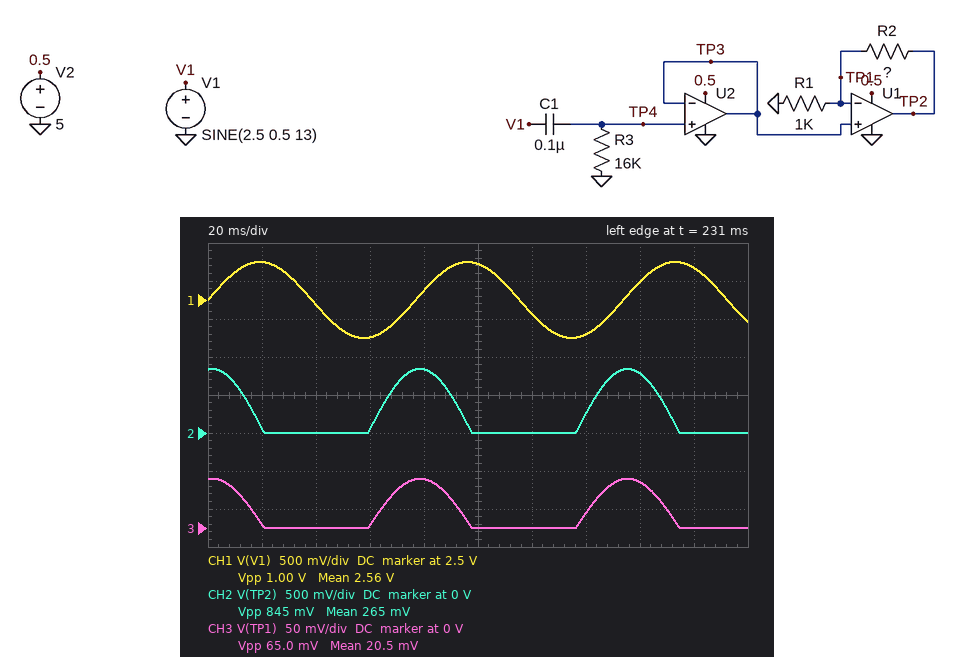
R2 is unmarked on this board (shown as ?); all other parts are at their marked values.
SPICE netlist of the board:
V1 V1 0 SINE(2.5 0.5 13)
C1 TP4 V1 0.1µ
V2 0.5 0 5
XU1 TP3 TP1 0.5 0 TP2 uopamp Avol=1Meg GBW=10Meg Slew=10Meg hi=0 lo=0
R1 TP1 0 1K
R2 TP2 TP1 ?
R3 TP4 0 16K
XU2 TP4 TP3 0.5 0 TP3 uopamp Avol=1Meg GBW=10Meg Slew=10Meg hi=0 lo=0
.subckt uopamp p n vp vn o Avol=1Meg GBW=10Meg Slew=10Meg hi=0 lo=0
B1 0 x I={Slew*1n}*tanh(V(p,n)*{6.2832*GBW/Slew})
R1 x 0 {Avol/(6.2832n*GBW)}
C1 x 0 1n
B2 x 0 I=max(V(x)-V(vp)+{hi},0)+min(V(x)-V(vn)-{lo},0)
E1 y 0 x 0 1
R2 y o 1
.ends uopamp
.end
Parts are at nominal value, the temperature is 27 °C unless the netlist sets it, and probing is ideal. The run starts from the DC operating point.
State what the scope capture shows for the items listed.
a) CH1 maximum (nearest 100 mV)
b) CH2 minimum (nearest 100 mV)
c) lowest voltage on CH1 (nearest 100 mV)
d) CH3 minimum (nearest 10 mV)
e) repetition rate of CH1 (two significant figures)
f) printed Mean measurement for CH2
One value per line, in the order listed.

3.0 V
0 V
2.0 V
0 V
13 Hz
265 mV
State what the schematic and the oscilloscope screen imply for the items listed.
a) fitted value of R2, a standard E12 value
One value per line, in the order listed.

12 kΩ
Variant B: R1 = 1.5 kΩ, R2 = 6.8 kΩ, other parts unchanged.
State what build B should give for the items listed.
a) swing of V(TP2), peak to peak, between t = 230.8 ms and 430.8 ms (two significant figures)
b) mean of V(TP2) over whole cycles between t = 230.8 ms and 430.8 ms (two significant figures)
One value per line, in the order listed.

360 mV
110 mV
